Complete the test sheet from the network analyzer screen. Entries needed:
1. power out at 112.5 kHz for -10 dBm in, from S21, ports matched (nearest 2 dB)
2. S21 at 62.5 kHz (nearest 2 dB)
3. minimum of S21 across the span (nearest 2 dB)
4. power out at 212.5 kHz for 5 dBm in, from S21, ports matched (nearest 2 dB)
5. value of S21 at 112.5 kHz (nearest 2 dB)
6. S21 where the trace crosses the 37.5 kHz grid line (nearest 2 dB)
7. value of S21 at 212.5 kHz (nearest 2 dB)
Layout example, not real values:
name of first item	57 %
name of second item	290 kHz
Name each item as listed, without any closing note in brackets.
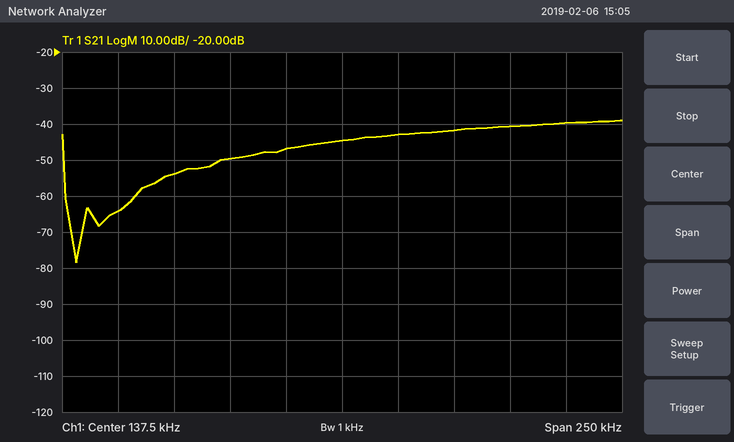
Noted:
power out at 112.5 kHz for -10 dBm in, from S21, ports matched	-56 dBm
S21 at 62.5 kHz	-54 dB
minimum of S21 across the span	-78 dB
power out at 212.5 kHz for 5 dBm in, from S21, ports matched	-36 dBm
value of S21 at 112.5 kHz	-46 dB
S21 where the trace crosses the 37.5 kHz grid line	-64 dB
value of S21 at 212.5 kHz	-40 dB
